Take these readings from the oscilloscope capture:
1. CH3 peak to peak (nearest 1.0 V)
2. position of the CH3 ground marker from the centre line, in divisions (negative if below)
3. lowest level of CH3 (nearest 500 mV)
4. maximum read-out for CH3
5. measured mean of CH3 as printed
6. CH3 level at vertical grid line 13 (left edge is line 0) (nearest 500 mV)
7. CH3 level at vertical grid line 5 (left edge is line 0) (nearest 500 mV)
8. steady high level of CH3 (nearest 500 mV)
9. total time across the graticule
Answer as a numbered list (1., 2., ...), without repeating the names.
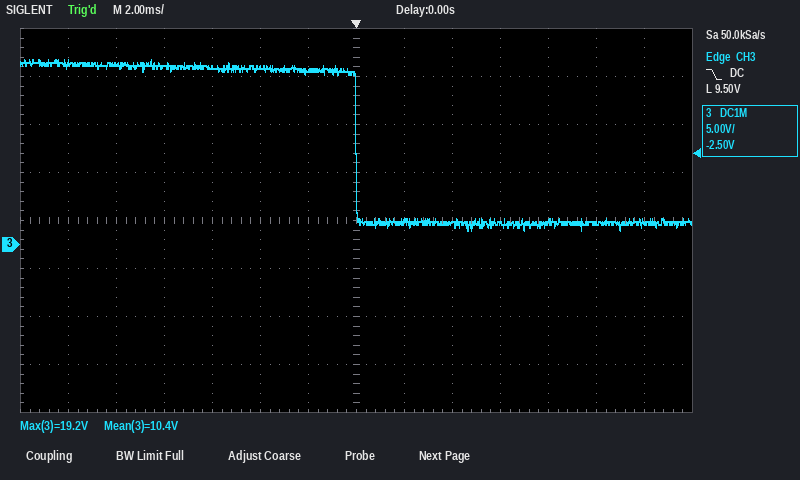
1. 18.0 V
2. -0.5 div
3. 1.5 V
4. 19.2 V
5. 10.4 V
6. 2.5 V
7. 18.5 V
8. 18.5 V
9. 28 ms
